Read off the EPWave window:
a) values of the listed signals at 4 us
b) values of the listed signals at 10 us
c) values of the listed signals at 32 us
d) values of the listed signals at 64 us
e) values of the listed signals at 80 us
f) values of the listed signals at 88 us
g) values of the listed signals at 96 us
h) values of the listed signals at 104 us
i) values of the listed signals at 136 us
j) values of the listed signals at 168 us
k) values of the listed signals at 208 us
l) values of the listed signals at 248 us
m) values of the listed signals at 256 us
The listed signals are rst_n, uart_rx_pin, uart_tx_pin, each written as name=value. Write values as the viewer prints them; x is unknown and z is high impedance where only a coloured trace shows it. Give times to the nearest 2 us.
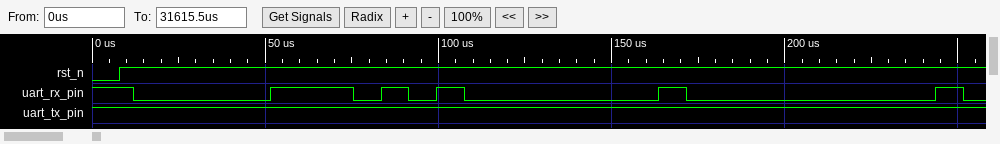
rst_n=0, uart_rx_pin=1, uart_tx_pin=1
rst_n=1, uart_rx_pin=1, uart_tx_pin=1
rst_n=1, uart_rx_pin=0, uart_tx_pin=1
rst_n=1, uart_rx_pin=1, uart_tx_pin=1
rst_n=1, uart_rx_pin=0, uart_tx_pin=1
rst_n=1, uart_rx_pin=1, uart_tx_pin=1
rst_n=1, uart_rx_pin=0, uart_tx_pin=1
rst_n=1, uart_rx_pin=1, uart_tx_pin=1
rst_n=1, uart_rx_pin=0, uart_tx_pin=1
rst_n=1, uart_rx_pin=1, uart_tx_pin=1
rst_n=1, uart_rx_pin=0, uart_tx_pin=1
rst_n=1, uart_rx_pin=1, uart_tx_pin=1
rst_n=1, uart_rx_pin=0, uart_tx_pin=1
